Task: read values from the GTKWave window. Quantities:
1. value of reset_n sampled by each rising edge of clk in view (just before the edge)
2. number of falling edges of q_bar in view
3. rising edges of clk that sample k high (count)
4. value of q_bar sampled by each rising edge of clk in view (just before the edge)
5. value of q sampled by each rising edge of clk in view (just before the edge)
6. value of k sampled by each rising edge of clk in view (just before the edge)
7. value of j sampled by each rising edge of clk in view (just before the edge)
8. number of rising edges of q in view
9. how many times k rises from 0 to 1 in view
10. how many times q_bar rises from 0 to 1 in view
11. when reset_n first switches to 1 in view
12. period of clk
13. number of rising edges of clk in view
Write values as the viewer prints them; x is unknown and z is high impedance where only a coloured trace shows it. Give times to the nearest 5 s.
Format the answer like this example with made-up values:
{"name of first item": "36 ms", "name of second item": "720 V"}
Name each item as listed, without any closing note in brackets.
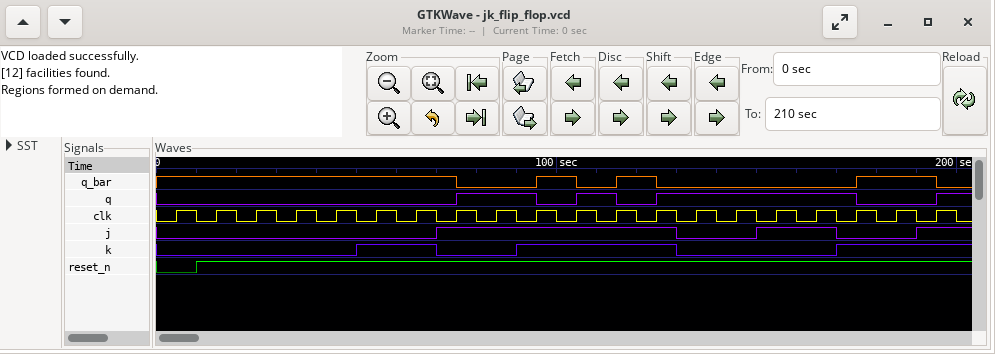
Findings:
{"value of reset_n sampled by each rising edge of clk in view": "0 1 1 1 1 1 1 1 1 1 1 1 1 1 1 1 1 1 1 1", "number of falling edges of q_bar in view": "4", "rising edges of clk that sample k high": "9", "value of q_bar sampled by each rising edge of clk in view": "1 1 1 1 1 1 1 1 0 0 1 0 1 0 0 0 0 0 1 1", "value of q sampled by each rising edge of clk in view": "0 0 0 0 0 0 0 0 1 1 0 1 0 1 1 1 1 1 0 0", "value of k sampled by each rising edge of clk in view": "0 0 0 0 0 1 1 0 0 1 1 1 1 0 0 0 0 1 1 1", "value of j sampled by each rising edge of clk in view": "0 0 0 0 0 0 0 1 1 1 1 1 1 0 0 1 1 0 0 1", "number of rising edges of q in view": "4", "how many times k rises from 0 to 1 in view": "3", "how many times q_bar rises from 0 to 1 in view": "3", "when reset_n first switches to 1 in view": "10 s", "period of clk": "10 s", "number of rising edges of clk in view": "20"}
